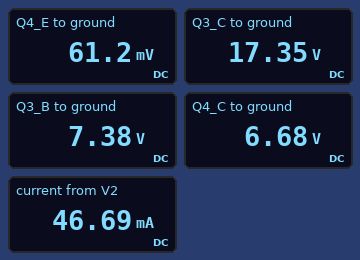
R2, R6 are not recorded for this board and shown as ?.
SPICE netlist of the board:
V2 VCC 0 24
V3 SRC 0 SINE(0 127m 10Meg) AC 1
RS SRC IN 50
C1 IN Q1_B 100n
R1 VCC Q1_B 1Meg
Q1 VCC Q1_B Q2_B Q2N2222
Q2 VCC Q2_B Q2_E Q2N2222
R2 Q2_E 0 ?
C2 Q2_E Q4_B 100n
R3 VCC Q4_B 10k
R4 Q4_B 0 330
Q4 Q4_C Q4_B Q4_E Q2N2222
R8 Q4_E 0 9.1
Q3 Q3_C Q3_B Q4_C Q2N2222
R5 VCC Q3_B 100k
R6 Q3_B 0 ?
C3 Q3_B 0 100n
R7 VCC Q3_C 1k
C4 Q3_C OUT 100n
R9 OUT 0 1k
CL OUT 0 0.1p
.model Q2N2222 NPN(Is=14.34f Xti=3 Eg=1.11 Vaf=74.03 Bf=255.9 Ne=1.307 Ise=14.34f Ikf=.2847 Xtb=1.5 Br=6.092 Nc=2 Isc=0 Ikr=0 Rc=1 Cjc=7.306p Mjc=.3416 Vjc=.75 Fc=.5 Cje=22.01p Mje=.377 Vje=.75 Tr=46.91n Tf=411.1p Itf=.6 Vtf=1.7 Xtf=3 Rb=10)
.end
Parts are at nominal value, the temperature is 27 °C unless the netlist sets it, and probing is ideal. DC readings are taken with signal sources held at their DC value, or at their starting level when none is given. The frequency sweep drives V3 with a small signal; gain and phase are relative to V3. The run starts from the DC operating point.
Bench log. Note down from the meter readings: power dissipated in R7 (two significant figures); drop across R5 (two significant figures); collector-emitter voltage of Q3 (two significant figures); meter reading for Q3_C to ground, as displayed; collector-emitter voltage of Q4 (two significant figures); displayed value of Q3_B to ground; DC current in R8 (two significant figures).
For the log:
44 mW
17 V
11 V
17.35 V
6.6 V
7.38 V
6.7 mA
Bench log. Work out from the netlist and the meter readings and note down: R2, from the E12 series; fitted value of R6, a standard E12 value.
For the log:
560 Ω
56 kΩ
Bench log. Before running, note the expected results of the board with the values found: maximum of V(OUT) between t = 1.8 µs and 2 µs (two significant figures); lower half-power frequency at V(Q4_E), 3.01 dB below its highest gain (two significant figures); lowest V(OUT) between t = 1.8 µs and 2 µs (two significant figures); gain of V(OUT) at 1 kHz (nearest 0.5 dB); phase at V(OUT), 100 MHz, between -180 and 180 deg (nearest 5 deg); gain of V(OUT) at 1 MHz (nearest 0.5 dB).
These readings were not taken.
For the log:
3.1 V
5.6 kHz
-5.3 V
14.5 dB
30 deg
31.5 dB
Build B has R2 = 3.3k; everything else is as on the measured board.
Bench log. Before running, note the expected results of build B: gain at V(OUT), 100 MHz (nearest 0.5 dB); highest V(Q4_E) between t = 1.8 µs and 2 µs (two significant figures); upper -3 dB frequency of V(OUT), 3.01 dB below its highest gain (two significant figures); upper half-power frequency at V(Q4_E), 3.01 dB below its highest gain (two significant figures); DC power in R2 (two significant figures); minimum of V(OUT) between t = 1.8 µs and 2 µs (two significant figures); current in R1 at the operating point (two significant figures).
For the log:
22.0 dB
150 mV
46 MHz
66 MHz
150 mW
-4.8 V
380 nA
